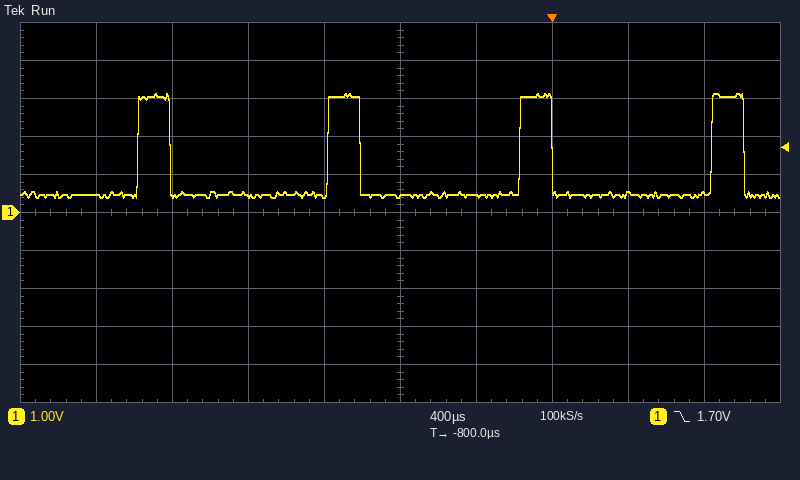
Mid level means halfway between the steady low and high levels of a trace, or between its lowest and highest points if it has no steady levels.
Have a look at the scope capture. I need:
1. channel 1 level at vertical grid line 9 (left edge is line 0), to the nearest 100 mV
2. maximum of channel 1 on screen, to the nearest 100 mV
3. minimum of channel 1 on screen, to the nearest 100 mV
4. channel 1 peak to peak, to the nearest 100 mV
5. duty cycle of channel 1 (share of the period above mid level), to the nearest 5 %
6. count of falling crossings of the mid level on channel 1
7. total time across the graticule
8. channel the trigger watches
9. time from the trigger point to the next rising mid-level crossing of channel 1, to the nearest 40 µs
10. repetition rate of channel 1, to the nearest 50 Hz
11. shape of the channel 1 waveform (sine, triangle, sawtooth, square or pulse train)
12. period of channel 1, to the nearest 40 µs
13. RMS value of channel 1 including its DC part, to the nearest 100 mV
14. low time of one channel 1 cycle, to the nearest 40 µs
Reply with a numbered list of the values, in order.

1. 500 mV
2. 3.1 V
3. 400 mV
4. 2.7 V
5. 15 %
6. 4
7. 4 ms
8. channel 1
9. 840 µs
10. 1.00 kHz
11. pulse train
12. 1.00 ms
13. 1.3 V
14. 840 µs
